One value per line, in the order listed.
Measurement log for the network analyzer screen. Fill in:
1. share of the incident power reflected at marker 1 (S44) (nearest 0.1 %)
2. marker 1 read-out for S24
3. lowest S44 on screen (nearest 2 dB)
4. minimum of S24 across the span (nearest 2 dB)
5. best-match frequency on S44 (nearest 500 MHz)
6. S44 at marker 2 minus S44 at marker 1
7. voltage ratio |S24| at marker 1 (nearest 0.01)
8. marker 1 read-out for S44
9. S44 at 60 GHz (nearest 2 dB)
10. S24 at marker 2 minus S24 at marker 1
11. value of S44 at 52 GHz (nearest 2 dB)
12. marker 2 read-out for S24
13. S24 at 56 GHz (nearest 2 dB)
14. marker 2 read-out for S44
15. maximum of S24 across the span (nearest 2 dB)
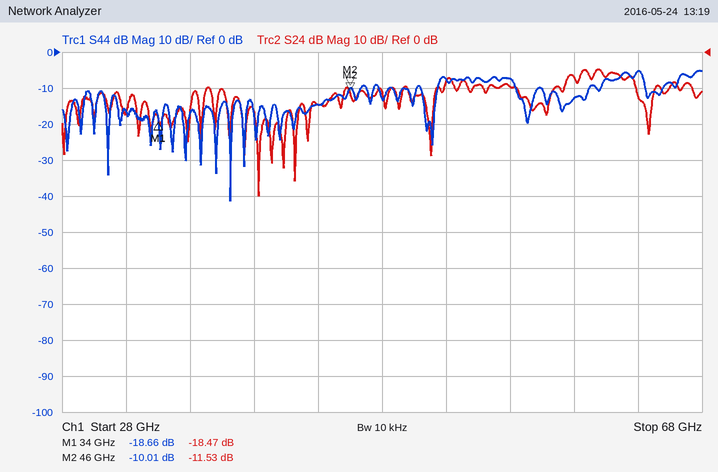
1.4 %
-18.47 dB
-42 dB
-40 dB
38.5 GHz
8.65 dB
0.12
-18.66 dB
-12 dB
6.94 dB
-8 dB
-11.53 dB
-10 dB
-10.01 dB
-4 dB
